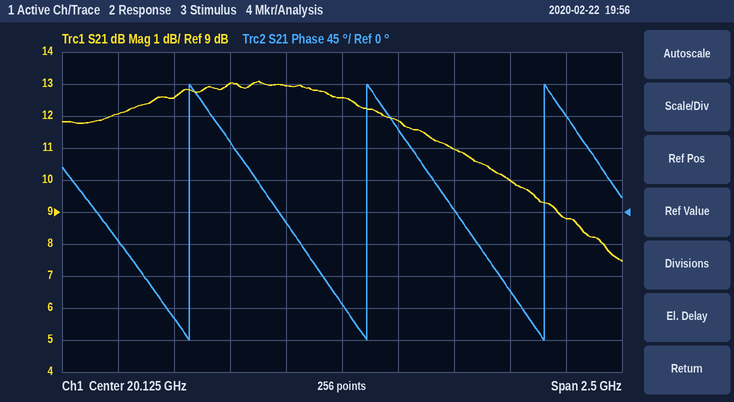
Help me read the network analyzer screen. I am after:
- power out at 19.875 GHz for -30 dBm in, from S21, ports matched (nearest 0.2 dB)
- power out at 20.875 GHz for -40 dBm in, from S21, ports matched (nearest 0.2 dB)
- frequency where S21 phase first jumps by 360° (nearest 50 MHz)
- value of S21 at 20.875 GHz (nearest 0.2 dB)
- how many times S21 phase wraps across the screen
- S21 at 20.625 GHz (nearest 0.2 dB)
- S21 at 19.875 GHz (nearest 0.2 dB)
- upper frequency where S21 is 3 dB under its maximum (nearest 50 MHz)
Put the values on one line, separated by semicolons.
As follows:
-17.0 dBm; -30.0 dBm; 19.45 GHz; 10.0 dB; 3; 11.0 dB; 13.0 dB; 20.85 GHz
